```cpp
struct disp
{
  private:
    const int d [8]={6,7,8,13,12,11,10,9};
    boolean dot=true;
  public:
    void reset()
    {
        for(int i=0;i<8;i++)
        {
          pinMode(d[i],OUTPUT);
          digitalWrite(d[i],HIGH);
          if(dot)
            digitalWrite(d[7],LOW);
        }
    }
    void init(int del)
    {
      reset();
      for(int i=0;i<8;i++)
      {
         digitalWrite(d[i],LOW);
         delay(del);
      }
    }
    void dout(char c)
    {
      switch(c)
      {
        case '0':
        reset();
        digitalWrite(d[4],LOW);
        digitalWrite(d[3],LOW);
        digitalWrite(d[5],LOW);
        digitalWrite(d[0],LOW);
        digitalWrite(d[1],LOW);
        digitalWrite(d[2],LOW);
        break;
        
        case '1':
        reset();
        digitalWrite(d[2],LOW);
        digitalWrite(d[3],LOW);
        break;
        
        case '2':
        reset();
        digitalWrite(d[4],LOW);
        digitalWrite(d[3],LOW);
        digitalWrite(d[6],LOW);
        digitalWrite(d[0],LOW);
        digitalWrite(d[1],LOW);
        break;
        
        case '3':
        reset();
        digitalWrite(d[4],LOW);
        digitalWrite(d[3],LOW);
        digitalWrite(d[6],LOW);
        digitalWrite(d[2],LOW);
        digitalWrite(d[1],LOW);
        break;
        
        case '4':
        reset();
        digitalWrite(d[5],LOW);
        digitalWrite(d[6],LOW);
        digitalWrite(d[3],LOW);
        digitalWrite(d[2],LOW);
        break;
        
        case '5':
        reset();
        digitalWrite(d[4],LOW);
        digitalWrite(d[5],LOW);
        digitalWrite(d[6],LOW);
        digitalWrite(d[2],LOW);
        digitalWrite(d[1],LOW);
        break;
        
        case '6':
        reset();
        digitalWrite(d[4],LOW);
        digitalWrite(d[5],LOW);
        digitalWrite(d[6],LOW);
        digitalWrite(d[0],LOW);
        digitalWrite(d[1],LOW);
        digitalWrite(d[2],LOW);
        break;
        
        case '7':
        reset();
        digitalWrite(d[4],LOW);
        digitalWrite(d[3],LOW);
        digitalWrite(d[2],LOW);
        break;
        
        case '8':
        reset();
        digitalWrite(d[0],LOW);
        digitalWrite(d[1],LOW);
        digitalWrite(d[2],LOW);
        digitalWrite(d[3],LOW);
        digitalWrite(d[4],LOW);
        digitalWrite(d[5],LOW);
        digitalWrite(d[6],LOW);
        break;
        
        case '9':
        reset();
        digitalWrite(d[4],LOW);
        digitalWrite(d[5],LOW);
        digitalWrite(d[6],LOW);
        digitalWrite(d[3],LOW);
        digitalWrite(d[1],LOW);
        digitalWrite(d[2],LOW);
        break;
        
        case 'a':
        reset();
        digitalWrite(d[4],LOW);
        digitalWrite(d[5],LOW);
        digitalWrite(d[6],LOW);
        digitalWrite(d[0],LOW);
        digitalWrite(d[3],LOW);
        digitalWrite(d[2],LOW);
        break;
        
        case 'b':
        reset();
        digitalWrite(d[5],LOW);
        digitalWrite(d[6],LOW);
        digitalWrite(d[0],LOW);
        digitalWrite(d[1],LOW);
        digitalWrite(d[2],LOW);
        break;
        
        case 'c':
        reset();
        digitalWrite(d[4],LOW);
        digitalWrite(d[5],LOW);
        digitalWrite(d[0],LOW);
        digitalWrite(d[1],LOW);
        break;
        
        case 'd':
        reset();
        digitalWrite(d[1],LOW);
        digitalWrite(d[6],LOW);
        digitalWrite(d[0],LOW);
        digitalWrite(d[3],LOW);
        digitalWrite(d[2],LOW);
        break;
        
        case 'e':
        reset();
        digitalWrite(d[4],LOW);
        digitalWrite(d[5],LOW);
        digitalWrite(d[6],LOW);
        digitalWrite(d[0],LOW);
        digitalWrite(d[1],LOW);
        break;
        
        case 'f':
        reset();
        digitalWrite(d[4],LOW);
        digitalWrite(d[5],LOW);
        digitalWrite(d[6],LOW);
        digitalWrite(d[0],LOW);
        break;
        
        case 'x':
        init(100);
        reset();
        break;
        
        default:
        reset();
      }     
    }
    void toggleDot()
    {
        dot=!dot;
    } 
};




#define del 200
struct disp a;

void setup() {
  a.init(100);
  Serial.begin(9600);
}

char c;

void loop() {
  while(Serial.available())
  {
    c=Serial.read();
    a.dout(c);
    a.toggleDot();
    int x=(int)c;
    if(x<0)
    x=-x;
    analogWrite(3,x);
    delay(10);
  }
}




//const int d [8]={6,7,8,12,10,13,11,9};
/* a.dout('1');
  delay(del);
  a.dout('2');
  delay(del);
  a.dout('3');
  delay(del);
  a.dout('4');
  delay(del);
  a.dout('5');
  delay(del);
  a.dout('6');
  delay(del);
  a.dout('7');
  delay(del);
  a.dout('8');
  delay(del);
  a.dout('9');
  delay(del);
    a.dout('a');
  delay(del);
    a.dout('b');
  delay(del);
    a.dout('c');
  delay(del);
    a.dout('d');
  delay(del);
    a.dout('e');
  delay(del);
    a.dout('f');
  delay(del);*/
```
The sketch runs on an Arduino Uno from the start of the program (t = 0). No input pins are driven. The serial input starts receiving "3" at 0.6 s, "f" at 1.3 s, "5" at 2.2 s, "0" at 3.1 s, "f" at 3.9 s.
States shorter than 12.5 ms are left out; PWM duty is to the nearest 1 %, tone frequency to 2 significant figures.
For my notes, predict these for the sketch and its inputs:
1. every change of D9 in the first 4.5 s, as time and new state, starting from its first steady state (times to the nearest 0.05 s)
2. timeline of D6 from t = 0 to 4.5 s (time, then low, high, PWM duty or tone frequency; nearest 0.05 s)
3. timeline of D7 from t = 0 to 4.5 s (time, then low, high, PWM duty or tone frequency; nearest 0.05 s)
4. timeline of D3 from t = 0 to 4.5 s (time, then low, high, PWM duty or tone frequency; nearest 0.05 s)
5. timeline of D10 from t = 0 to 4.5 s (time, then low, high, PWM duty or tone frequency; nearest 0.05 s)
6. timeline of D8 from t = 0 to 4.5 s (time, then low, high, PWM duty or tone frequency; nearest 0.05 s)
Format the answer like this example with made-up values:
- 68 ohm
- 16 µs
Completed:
- 0 s low; 2.2 s high; 3.1 s low; 3.9 s high
- 0 s low; 2.2 s high; 3.1 s low
- 0 s high; 0.1 s low; 1.3 s high; 2.2 s low; 3.9 s high
- 1.3 s PWM 40 %; 2.2 s PWM 21 %; 3.1 s PWM 19 %; 3.9 s PWM 40 %
- 0 s high; 0.6 s low; 3.1 s high; 3.9 s low
- 0 s high; 0.2 s low; 1.3 s high; 2.2 s low; 3.9 s high
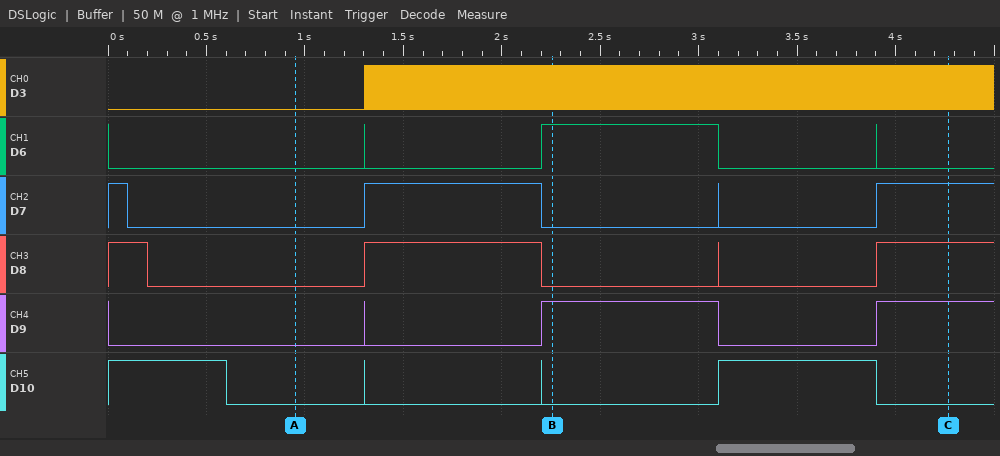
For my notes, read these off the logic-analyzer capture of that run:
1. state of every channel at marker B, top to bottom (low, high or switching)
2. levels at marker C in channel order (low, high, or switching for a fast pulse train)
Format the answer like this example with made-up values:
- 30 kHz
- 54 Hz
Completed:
- D3 switching, D6 high, D7 low, D8 low, D9 high, D10 low
- D3 switching, D6 low, D7 high, D8 high, D9 high, D10 low
